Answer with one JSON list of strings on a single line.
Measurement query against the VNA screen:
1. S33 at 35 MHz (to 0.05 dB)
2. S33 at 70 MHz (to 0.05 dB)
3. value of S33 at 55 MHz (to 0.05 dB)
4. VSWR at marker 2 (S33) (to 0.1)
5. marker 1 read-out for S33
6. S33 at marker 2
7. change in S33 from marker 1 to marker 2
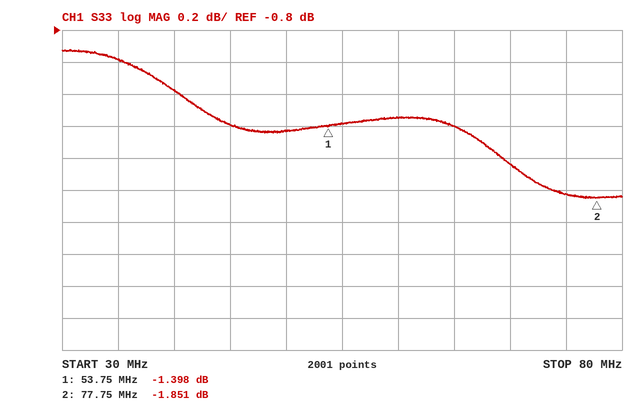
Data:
["-1.00 dB", "-1.65 dB", "-1.40 dB", "9.4", "-1.398 dB", "-1.851 dB", "-0.453 dB"]
